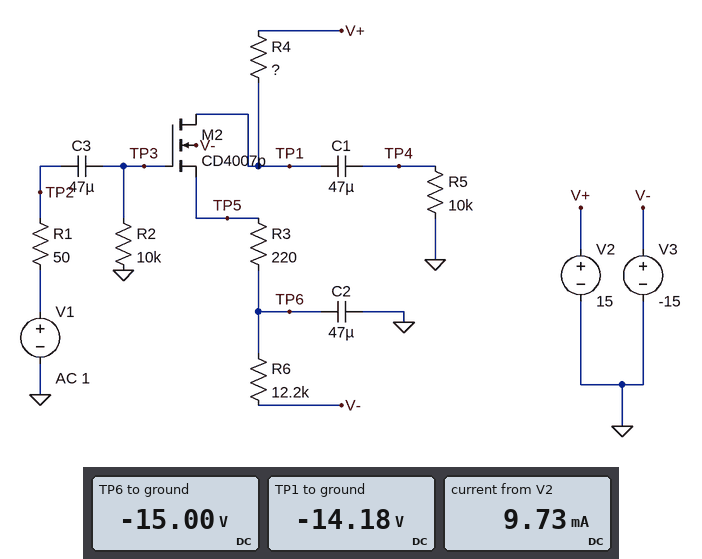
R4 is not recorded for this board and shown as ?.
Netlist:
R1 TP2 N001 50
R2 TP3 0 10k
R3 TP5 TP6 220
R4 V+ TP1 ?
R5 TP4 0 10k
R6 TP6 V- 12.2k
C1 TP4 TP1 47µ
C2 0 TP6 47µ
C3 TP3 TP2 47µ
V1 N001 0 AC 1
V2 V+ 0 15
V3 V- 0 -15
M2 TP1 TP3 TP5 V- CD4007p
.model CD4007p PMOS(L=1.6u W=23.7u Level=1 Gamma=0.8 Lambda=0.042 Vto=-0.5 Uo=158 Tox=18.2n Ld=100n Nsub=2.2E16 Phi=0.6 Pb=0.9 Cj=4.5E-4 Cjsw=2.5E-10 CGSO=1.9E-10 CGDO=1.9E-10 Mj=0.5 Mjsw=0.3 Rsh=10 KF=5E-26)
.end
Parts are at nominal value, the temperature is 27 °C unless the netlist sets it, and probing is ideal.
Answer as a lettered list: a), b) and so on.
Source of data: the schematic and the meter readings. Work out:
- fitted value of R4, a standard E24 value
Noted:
a) 3 kΩ
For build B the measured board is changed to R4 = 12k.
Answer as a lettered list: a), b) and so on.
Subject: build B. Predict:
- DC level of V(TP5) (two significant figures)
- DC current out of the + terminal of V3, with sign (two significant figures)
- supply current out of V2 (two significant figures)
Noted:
a) -15 V
b) -2.4 mA
c) 2.4 mA
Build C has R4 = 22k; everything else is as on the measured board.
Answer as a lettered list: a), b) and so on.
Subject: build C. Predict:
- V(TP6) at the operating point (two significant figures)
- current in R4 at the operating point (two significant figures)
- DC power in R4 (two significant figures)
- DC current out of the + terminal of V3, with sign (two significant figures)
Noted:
a) -15 V
b) 1.3 mA
c) 39 mW
d) -1.3 mA
